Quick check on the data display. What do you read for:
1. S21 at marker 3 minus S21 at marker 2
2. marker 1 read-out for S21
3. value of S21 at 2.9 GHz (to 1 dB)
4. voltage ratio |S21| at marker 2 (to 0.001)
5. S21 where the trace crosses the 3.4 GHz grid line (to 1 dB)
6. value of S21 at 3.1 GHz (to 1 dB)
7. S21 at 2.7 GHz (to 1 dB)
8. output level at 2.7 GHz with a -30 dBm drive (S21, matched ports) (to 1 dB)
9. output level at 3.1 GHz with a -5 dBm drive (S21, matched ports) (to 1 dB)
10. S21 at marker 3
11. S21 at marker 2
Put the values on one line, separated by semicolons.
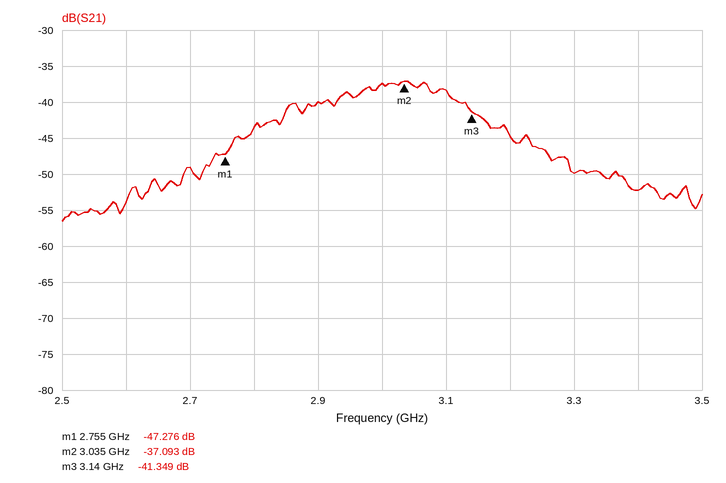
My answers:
-4.256 dB; -47.276 dB; -40 dB; 0.014; -52 dB; -38 dB; -49 dB; -79 dBm; -43 dBm; -41.349 dB; -37.093 dB
